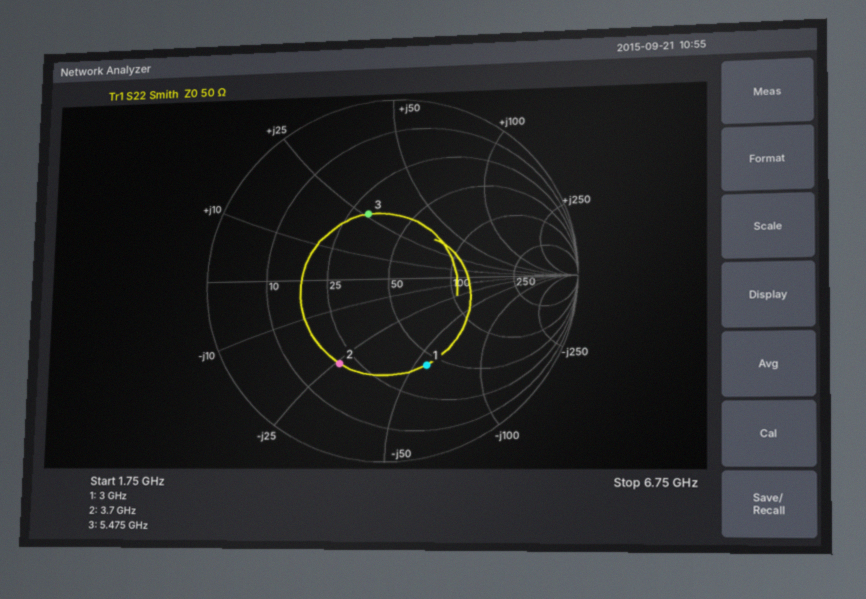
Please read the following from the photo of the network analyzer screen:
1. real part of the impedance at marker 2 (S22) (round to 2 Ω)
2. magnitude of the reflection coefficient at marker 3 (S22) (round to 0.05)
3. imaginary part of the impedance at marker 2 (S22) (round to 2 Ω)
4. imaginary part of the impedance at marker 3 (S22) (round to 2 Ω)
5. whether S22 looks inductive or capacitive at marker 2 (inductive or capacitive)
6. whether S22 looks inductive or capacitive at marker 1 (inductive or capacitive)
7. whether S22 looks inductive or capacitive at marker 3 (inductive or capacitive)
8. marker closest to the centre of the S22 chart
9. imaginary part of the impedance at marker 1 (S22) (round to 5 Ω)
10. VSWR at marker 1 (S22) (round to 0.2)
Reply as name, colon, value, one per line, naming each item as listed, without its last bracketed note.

real part of the impedance at marker 2 (S22): 20 Ω
magnitude of the reflection coefficient at marker 3 (S22): 0.40
imaginary part of the impedance at marker 2 (S22): -26 Ω
imaginary part of the impedance at marker 3 (S22): +26 Ω
whether S22 looks inductive or capacitive at marker 2: capacitive
whether S22 looks inductive or capacitive at marker 1: capacitive
whether S22 looks inductive or capacitive at marker 3: inductive
marker closest to the centre of the S22 chart: marker 3
imaginary part of the impedance at marker 1 (S22): -55 Ω
VSWR at marker 1 (S22): 3.2
